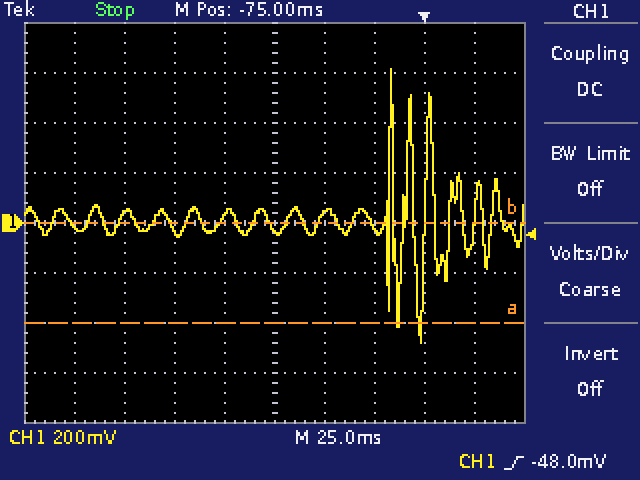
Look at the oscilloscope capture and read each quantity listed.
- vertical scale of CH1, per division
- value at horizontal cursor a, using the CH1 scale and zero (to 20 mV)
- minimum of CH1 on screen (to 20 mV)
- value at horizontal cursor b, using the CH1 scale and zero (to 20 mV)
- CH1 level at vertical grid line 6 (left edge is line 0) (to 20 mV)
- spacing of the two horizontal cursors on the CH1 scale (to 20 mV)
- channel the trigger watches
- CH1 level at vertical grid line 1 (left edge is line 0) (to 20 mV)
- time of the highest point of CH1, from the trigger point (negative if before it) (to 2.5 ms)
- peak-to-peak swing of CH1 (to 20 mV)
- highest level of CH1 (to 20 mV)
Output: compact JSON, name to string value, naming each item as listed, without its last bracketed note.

{"vertical scale of CH1, per division": "200 mV", "value at horizontal cursor a, using the CH1 scale and zero": "-400 mV", "minimum of CH1 on screen": "-480 mV", "value at horizontal cursor b, using the CH1 scale and zero": "0 mV", "CH1 level at vertical grid line 6 (left edge is line 0)": "40 mV", "spacing of the two horizontal cursors on the CH1 scale": "400 mV", "channel the trigger watches": "CH1", "CH1 level at vertical grid line 1 (left edge is line 0)": "-20 mV", "time of the highest point of CH1, from the trigger point (negative if before it)": "-17.5 ms", "peak-to-peak swing of CH1": "1.10 V", "highest level of CH1": "620 mV"}
